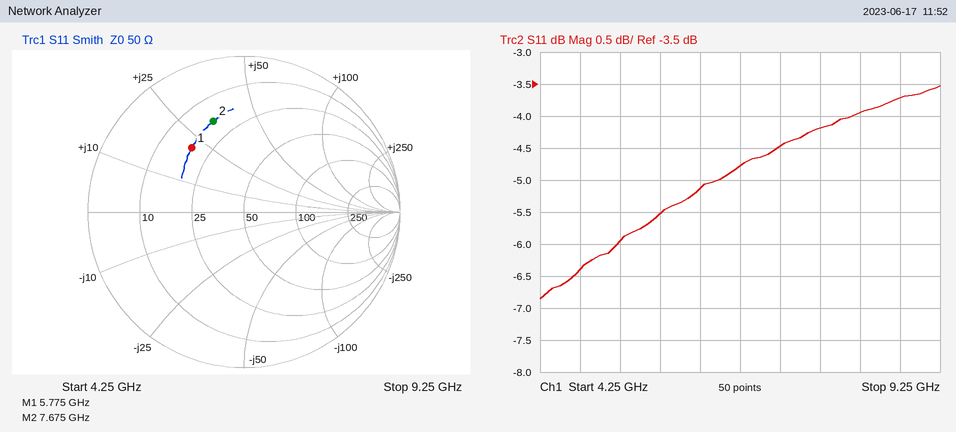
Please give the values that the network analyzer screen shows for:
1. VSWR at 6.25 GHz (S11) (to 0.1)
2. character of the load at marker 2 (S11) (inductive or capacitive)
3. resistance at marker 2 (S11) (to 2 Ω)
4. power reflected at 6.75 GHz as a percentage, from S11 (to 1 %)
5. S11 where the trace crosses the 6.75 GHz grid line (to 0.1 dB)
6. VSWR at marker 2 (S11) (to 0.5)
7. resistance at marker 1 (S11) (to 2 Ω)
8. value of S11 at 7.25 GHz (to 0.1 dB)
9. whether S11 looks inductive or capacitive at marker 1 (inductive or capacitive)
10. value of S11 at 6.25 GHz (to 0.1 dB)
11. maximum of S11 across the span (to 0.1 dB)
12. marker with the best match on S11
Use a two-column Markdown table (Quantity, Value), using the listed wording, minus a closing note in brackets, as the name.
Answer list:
| Quantity | Value |
|---|---|
| VSWR at 6.25 GHz (S11) | 3.5 |
| character of the load at marker 2 (S11) | inductive |
| resistance at marker 2 (S11) | 18 Ω |
| power reflected at 6.75 GHz as a percentage, from S11 | 33 % |
| S11 where the trace crosses the 6.75 GHz grid line | -4.8 dB |
| VSWR at marker 2 (S11) | 4.0 |
| resistance at marker 1 (S11) | 18 Ω |
| value of S11 at 7.25 GHz | -4.5 dB |
| whether S11 looks inductive or capacitive at marker 1 | inductive |
| value of S11 at 6.25 GHz | -5.1 dB |
| maximum of S11 across the span | -3.5 dB |
| marker with the best match on S11 | marker 1 |
